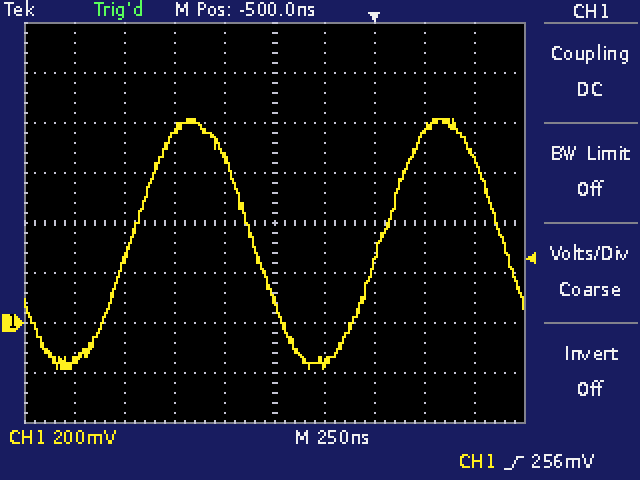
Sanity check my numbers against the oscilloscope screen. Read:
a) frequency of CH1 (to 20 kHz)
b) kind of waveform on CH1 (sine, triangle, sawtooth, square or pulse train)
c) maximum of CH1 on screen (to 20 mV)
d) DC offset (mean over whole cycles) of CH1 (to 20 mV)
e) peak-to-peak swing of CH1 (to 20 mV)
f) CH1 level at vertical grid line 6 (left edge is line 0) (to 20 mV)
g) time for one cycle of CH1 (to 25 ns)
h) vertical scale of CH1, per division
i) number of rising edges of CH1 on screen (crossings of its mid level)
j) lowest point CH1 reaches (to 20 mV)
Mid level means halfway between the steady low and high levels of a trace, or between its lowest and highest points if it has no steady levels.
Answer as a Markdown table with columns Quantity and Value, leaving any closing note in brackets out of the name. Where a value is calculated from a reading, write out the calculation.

| Quantity | Value |
|---|---|
| frequency of CH1 | 1 / 1.250 µs ≈ 800 kHz |
| kind of waveform on CH1 | sine |
| maximum of CH1 on screen | 820 mV |
| DC offset (mean over whole cycles) of CH1 | (820 mV + (-180 mV)) / 2 ≈ 320 mV |
| peak-to-peak swing of CH1 | 820 mV − (-180 mV) = 1.00 V |
| CH1 level at vertical grid line 6 (left edge is line 0) | -160 mV |
| time for one cycle of CH1 | 1.250 µs |
| vertical scale of CH1, per division | 200 mV |
| number of rising edges of CH1 on screen | 2 |
| lowest point CH1 reaches | -180 mV |
